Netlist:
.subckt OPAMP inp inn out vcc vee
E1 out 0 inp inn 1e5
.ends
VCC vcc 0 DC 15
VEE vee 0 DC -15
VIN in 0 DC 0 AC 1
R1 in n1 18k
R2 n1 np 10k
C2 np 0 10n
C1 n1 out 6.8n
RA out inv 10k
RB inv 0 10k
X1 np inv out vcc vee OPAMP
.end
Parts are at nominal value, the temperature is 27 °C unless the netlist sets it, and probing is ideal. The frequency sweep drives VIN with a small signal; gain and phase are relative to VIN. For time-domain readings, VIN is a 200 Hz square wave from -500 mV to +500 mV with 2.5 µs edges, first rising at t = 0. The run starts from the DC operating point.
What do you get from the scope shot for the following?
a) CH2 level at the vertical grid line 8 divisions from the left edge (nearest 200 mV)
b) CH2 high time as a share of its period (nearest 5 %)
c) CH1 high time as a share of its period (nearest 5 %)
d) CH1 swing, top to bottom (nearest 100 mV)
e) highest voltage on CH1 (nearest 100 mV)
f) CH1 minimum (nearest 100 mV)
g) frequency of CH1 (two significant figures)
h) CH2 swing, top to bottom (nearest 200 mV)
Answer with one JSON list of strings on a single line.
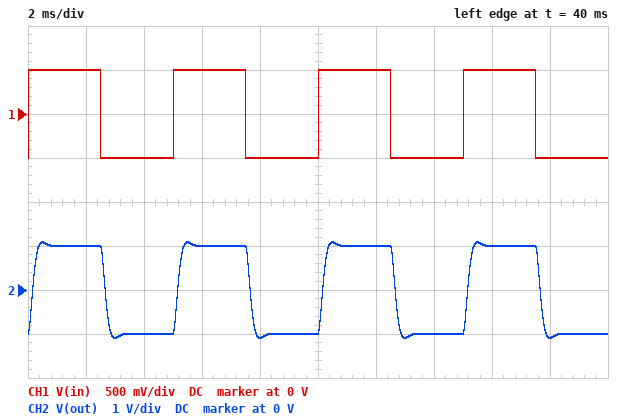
["1.0 V", "50 %", "50 %", "1.0 V", "500 mV", "-500 mV", "200 Hz", "2.2 V"]
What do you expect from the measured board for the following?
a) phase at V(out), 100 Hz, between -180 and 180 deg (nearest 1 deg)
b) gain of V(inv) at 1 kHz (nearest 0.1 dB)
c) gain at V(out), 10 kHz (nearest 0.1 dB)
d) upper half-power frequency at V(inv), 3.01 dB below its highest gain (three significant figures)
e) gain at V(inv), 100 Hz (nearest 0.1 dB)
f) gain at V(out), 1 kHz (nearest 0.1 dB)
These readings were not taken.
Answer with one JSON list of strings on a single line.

["-6 deg", "-1.0 dB", "-27.7 dB", "1.43 kHz", "0 dB", "5.1 dB"]
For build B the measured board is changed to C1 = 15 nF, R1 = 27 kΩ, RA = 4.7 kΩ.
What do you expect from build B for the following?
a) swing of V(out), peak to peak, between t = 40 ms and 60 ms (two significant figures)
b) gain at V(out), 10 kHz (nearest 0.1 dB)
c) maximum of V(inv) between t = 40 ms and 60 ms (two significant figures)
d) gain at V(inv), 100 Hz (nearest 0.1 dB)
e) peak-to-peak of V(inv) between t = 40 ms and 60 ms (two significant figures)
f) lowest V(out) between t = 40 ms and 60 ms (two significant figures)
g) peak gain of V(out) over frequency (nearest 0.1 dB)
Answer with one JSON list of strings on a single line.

["2.1 V", "-40.7 dB", "710 mV", "0.1 dB", "1.4 V", "-1.0 V", "5.3 dB"]
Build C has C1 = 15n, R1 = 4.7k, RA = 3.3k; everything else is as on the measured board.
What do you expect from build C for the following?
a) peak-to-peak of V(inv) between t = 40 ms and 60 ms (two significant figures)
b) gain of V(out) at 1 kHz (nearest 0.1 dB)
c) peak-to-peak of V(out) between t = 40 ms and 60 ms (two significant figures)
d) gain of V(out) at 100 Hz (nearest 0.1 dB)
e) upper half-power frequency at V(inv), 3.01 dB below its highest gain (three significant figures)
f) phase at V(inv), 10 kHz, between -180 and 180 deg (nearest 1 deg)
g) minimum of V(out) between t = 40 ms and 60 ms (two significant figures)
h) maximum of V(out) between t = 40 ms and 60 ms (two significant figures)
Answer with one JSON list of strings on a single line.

["1.1 V", "2.0 dB", "1.4 V", "2.5 dB", "1.82 kHz", "-164 deg", "-710 mV", "710 mV"]
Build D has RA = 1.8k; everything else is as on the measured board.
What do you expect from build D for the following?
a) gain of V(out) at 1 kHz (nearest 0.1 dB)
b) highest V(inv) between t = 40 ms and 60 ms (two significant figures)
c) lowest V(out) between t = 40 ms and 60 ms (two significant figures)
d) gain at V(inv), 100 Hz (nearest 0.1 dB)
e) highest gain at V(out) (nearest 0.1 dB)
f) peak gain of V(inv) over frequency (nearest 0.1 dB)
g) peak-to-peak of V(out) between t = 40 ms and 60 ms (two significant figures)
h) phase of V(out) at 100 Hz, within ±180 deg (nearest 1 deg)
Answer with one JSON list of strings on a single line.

["-3.2 dB", "500 mV", "-590 mV", "-0.1 dB", "1.4 dB", "0 dB", "1.2 V", "-9 deg"]
